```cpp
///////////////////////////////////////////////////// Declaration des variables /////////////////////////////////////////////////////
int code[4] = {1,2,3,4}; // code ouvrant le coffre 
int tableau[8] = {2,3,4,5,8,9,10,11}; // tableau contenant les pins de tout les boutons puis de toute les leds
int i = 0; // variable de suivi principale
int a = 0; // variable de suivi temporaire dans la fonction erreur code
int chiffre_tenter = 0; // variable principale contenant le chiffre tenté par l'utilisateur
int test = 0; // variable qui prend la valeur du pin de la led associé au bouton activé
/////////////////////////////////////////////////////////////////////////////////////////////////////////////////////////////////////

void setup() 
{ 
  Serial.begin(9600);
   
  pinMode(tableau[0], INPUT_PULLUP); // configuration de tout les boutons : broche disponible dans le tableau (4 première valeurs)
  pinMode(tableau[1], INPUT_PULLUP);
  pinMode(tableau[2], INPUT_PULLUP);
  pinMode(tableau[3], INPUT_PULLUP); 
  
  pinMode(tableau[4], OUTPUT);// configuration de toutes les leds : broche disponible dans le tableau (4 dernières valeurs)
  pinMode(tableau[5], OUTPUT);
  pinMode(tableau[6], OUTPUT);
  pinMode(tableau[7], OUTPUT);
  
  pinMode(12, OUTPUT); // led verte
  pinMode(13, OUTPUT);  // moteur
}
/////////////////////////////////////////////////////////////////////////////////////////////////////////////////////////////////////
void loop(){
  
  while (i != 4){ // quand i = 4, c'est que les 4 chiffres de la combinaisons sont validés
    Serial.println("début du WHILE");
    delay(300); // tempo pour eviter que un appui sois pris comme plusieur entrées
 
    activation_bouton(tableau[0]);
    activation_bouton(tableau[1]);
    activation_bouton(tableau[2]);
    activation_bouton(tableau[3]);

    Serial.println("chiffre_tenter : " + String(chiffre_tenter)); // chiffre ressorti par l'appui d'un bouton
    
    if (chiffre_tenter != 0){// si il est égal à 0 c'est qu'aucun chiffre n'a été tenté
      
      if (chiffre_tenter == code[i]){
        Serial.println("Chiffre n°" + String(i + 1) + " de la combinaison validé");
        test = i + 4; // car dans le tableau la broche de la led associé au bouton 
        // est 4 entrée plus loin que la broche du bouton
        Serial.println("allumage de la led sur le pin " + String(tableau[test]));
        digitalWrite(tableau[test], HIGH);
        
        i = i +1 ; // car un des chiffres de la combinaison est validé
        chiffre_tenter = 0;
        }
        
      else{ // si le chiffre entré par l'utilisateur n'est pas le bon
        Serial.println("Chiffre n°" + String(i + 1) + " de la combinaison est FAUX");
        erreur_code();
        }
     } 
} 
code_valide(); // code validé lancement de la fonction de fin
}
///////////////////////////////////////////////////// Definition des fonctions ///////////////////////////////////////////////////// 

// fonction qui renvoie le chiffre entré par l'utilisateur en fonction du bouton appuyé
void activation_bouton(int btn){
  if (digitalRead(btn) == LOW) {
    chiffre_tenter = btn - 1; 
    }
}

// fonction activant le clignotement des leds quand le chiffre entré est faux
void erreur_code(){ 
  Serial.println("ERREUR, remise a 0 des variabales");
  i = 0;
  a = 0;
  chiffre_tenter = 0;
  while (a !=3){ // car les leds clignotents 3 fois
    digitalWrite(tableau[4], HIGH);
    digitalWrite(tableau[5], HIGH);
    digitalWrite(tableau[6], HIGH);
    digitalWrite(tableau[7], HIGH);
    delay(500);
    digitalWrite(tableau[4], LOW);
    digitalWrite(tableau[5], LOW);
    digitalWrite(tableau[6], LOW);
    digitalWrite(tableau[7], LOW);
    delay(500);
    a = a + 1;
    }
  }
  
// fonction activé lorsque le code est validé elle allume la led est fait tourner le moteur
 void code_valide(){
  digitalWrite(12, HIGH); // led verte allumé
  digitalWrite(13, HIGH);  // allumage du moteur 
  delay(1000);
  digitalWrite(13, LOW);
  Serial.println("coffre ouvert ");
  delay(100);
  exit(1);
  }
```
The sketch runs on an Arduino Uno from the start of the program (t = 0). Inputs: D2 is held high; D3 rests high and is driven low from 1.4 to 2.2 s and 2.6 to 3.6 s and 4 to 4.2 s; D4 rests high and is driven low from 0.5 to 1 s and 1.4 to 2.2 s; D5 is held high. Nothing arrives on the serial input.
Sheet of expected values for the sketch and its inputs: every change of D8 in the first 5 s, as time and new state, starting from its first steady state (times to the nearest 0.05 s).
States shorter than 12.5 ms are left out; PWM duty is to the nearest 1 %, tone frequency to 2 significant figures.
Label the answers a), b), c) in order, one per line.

a) 0 s low; 0.65 s high; 1.15 s low; 1.65 s high; 2.15 s low; 2.65 s high; 3.15 s low
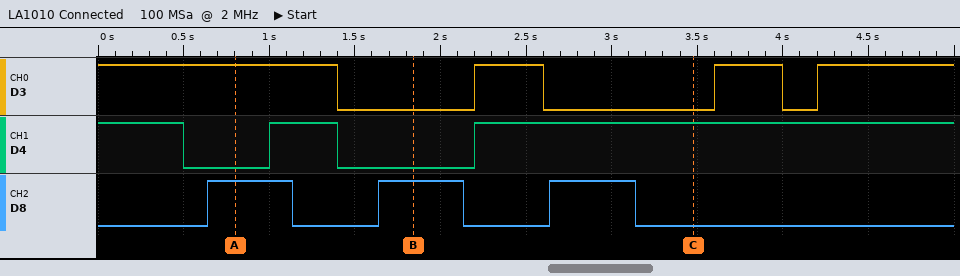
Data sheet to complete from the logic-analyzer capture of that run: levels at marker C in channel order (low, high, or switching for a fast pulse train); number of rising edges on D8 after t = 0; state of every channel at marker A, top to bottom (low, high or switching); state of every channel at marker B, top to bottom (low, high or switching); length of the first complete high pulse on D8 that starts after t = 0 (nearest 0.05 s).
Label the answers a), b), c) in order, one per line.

a) D3 low, D4 high, D8 low
b) 3
c) D3 high, D4 low, D8 high
d) D3 low, D4 low, D8 high
e) 0.50 s
